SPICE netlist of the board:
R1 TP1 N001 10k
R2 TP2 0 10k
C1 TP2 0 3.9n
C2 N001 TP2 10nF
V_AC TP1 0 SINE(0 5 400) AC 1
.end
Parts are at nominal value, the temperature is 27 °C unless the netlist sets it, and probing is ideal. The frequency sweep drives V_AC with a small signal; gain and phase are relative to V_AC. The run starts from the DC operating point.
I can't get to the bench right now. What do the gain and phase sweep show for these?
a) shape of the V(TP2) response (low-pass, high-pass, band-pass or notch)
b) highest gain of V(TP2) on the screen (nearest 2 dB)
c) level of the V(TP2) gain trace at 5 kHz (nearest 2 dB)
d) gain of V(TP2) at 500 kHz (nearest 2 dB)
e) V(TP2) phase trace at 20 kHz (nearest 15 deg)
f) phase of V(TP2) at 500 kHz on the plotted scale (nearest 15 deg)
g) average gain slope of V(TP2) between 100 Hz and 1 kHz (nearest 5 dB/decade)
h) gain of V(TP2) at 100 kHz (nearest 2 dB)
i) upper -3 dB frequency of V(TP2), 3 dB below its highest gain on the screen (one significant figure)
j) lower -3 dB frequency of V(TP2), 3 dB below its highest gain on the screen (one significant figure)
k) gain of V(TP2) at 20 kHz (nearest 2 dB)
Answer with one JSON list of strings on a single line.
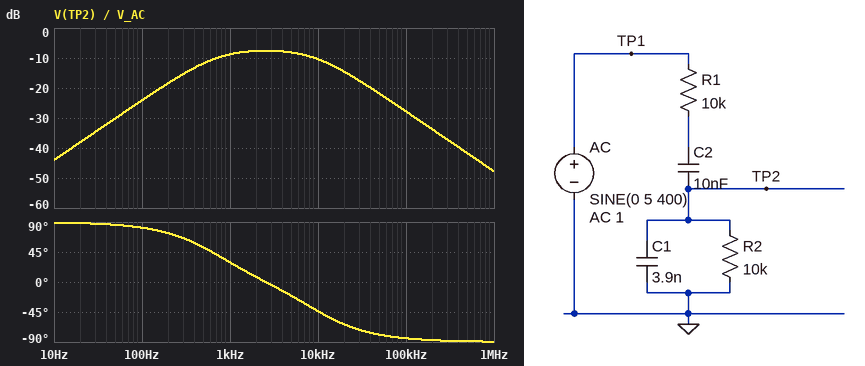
["band-pass", "-8 dB", "-8 dB", "-42 dB", "-60 deg", "-90 deg", "15 dB/decade", "-28 dB", "10 kHz", "600 Hz", "-14 dB"]
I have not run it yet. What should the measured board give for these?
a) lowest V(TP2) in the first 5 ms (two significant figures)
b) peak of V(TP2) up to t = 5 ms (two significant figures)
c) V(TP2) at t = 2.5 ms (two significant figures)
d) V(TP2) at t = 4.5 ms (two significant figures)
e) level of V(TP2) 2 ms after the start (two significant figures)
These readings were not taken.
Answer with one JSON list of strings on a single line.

["-1.1 V", "1.1 V", "930 mV", "-260 mV", "-260 mV"]
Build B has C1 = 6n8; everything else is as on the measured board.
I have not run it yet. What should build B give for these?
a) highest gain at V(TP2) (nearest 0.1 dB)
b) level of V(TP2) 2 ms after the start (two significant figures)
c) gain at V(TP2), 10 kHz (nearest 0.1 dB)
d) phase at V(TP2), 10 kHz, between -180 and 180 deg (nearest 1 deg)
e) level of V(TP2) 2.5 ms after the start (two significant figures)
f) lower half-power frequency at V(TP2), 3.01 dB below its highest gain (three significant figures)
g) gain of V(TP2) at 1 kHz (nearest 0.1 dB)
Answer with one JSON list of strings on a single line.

["-8.6 dB", "-320 mV", "-13.8 dB", "-57 deg", "880 mV", "546 Hz", "-9.3 dB"]
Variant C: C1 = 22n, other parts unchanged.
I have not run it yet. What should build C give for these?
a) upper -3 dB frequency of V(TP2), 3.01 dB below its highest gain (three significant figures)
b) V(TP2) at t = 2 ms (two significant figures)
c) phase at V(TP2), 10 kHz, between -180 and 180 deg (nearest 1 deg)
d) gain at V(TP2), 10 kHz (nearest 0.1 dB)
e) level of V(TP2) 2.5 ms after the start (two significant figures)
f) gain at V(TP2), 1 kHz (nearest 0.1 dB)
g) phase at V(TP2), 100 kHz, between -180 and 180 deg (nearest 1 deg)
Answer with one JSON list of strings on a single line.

["3.38 kHz", "-500 mV", "-73 deg", "-23.1 dB", "580 mV", "-12.5 dB", "-88 deg"]
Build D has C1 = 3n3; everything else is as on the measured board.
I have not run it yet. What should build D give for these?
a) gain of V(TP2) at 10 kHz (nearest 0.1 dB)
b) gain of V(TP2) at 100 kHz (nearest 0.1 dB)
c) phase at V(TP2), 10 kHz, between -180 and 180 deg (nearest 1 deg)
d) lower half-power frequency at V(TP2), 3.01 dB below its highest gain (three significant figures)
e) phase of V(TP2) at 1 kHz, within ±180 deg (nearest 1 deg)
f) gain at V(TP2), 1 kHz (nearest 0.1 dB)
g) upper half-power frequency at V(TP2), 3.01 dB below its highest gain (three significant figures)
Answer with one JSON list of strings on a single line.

["-9.6 dB", "-26.4 dB", "-39 deg", "646 Hz", "31 deg", "-8.7 dB", "11.9 kHz"]
